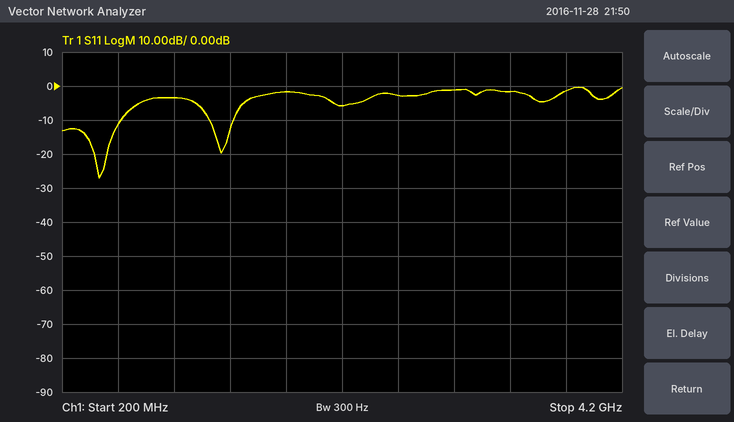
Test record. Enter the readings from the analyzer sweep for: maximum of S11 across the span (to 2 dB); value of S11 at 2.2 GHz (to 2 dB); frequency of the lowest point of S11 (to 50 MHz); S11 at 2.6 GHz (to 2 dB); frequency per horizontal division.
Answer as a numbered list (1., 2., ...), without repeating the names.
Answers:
1. 0 dB
2. -6 dB
3. 450 MHz
4. -2 dB
5. 400 MHz
